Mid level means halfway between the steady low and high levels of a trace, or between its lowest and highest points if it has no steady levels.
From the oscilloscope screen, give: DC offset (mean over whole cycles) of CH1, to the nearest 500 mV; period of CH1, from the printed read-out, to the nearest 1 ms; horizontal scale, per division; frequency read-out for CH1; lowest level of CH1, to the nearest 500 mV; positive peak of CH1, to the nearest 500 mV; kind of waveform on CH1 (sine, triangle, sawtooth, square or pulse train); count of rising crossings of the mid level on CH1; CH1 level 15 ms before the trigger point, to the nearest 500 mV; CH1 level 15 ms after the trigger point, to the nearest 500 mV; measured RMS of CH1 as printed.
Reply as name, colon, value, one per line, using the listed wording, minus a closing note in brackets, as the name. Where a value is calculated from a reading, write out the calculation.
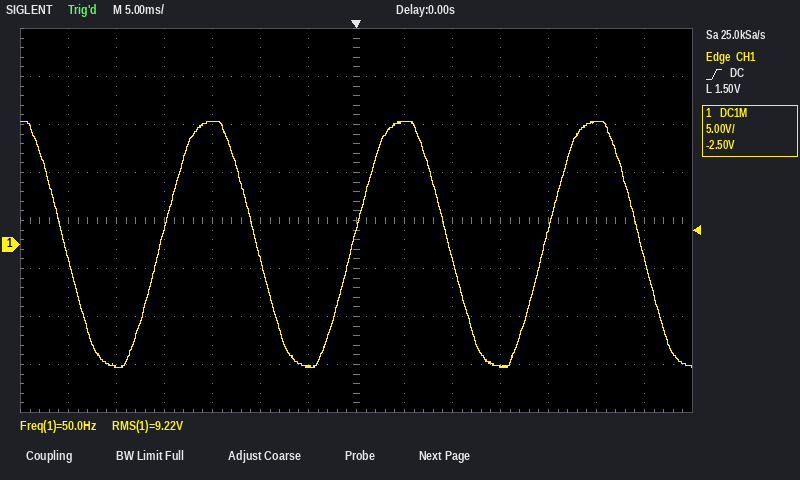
DC offset (mean over whole cycles) of CH1, to the nearest 500 mV: (13.0 V + (-13.0 V)) / 2 ≈ 0.0 V
period of CH1, from the printed read-out, to the nearest 1 ms: 1 / 50.0 Hz ≈ 20 ms
horizontal scale, per division: 5 ms
frequency read-out for CH1: 50.0 Hz
lowest level of CH1, to the nearest 500 mV: -13.0 V
positive peak of CH1, to the nearest 500 mV: 13.0 V
kind of waveform on CH1: sine
count of rising crossings of the mid level on CH1: 3
CH1 level 15 ms before the trigger point, to the nearest 500 mV: 13.0 V
CH1 level 15 ms after the trigger point, to the nearest 500 mV: -12.5 V
measured RMS of CH1 as printed: 9.22 V
